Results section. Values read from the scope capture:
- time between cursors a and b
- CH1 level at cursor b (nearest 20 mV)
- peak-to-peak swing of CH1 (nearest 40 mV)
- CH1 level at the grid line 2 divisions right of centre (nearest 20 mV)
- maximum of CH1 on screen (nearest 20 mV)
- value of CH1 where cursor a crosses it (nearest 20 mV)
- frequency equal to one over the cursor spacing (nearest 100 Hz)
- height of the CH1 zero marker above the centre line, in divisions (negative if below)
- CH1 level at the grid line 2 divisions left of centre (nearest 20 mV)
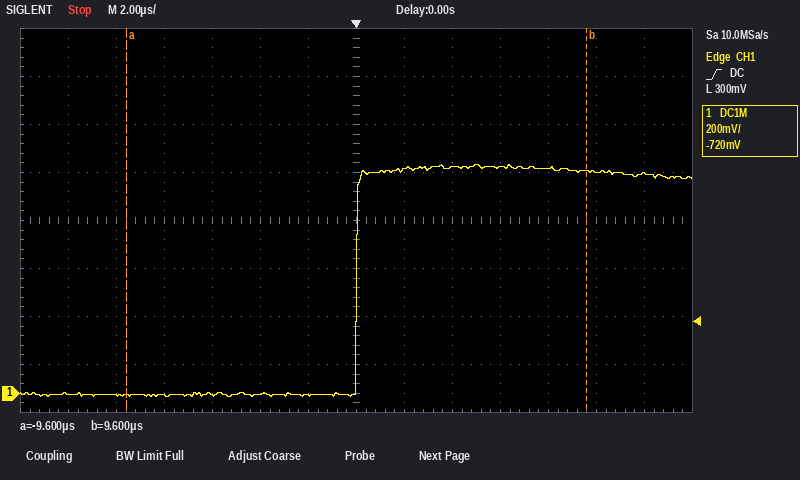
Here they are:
19.2 µs
920 mV
960 mV
940 mV
960 mV
0 mV
52.1 kHz
-3.6 div
0 mV
